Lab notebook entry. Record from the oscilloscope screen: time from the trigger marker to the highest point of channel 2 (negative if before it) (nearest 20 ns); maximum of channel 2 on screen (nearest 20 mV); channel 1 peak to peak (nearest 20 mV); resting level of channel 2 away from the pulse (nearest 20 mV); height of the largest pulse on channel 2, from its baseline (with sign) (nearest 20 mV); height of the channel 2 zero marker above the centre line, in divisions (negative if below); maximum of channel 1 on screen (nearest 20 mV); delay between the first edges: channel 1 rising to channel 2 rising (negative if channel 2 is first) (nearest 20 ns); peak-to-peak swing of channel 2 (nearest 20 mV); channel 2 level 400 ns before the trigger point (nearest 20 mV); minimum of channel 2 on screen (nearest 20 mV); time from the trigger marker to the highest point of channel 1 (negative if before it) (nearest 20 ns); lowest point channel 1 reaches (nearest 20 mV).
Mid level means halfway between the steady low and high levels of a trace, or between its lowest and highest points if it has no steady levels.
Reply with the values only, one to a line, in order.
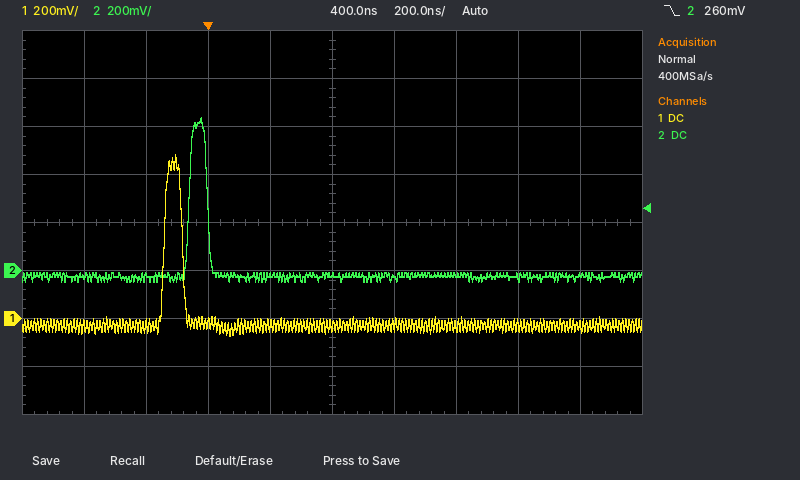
-20 ns
640 mV
760 mV
-20 mV
+660 mV
-1.0 div
680 mV
+80 ns
680 mV
-20 mV
-40 mV
-100 ns
-80 mV
